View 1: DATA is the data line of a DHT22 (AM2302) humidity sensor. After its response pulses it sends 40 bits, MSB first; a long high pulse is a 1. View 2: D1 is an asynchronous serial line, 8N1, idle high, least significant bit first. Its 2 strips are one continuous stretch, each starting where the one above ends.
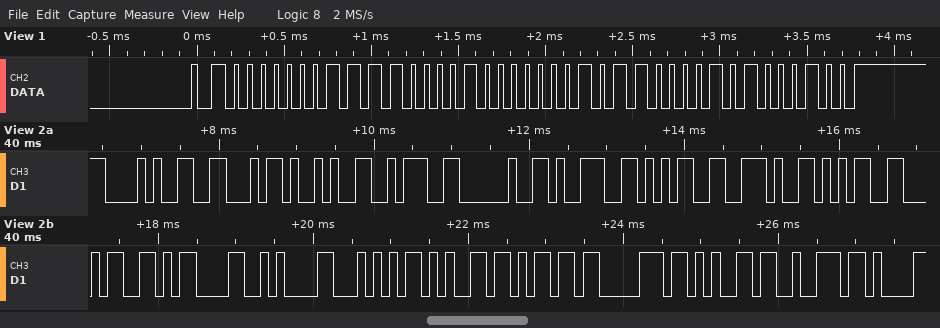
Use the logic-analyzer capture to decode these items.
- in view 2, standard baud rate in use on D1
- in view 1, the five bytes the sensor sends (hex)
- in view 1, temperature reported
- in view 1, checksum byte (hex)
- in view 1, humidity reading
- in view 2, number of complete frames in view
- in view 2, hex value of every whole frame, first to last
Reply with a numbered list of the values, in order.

1. 9600 baud
2. 01 E1 01 61 44
3. 35.3 °C
4. 0x44
5. 48.1 %
6. 18
7. 28 46 29 3A 20 39 35 2E 35 34 0D 0A 54 65 6D 70 65 72
